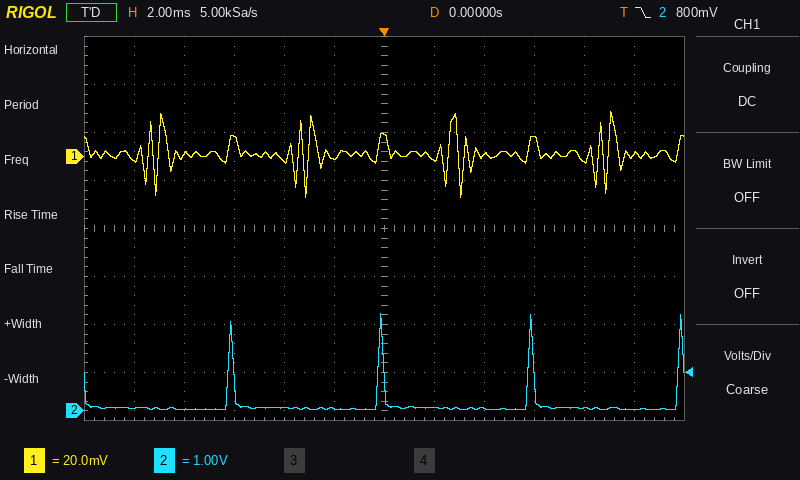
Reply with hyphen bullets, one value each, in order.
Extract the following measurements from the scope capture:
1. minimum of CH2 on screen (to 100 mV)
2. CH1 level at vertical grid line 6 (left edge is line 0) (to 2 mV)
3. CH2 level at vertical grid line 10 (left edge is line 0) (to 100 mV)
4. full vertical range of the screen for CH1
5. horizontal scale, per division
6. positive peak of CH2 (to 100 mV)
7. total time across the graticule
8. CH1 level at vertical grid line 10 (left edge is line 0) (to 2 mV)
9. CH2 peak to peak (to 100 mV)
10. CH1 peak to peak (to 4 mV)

- 0.0 V
- 8 mV
- 100 mV
- 160 mV
- 2 ms
- 2.0 V
- 24 ms
- -2 mV
- 2.0 V
- 36 mV
